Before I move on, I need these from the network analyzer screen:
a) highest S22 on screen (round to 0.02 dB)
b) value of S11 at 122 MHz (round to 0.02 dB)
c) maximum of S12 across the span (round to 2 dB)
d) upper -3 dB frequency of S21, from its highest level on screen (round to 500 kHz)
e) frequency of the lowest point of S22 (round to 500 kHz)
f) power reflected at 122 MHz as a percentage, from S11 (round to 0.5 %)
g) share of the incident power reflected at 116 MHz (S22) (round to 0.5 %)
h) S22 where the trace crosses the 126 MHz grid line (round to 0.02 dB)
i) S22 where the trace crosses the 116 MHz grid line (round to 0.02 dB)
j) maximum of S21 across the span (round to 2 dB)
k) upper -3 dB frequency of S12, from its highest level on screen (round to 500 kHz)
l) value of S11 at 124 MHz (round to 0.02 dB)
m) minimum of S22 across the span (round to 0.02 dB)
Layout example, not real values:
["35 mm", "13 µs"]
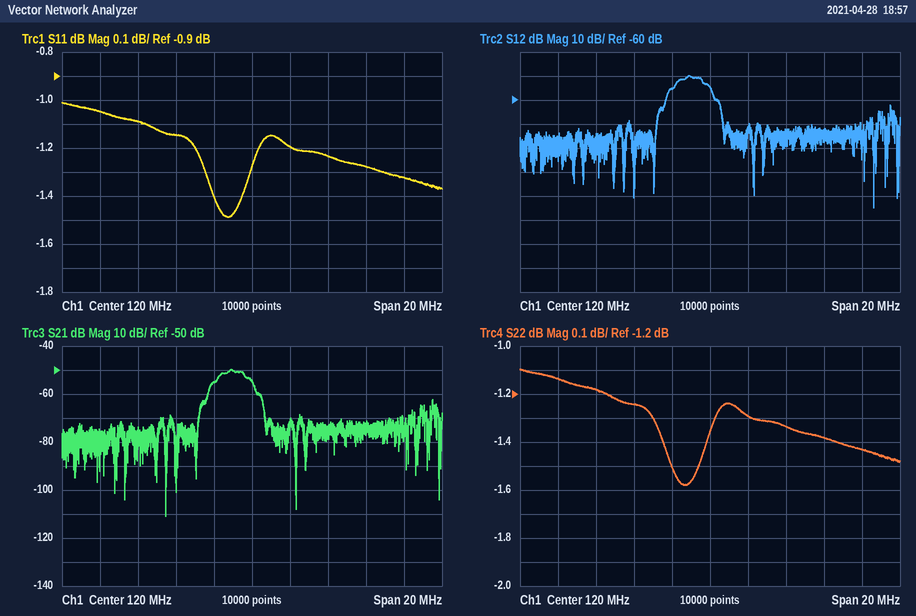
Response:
["-1.10 dB", "-1.20 dB", "-50 dB", "119.5 MHz", "118.5 MHz", "76.0 %", "75.0 %", "-1.38 dB", "-1.24 dB", "-50 dB", "119.5 MHz", "-1.24 dB", "-1.58 dB"]
